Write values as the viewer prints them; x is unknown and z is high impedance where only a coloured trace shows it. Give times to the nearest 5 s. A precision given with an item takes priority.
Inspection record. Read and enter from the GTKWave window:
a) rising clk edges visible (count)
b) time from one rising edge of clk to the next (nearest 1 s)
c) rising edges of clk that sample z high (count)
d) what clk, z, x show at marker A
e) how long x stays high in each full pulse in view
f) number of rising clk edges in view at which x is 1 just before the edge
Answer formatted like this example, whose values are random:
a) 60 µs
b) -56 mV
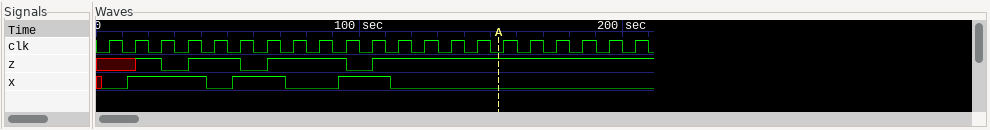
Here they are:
a) 21
b) 10 s
c) 16
d) clk=0, z=1, x=0
e) 30 s, 20 s, 20 s
f) 7
